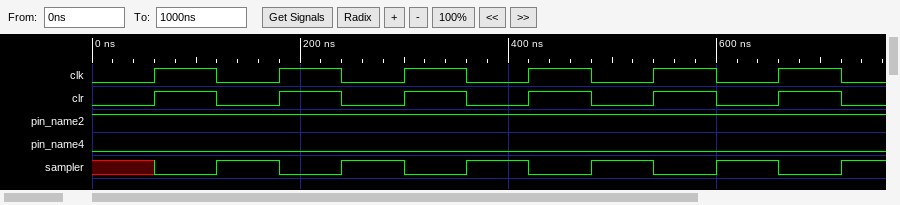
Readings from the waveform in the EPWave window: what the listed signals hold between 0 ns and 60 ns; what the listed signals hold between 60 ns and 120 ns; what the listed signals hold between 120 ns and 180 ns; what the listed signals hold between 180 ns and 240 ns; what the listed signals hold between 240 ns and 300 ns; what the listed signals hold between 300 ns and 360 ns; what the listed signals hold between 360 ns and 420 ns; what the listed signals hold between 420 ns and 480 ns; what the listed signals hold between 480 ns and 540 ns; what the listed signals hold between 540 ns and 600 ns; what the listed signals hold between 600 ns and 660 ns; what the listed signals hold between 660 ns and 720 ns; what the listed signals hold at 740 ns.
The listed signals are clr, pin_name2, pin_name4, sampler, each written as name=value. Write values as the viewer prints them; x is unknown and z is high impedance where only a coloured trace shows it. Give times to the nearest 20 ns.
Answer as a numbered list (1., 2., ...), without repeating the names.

1. clr=0, pin_name2=1, pin_name4=0, sampler=x
2. clr=1, pin_name2=1, pin_name4=0, sampler=0
3. clr=0, pin_name2=1, pin_name4=0, sampler=1
4. clr=1, pin_name2=1, pin_name4=0, sampler=0
5. clr=0, pin_name2=1, pin_name4=0, sampler=1
6. clr=1, pin_name2=1, pin_name4=0, sampler=0
7. clr=0, pin_name2=1, pin_name4=0, sampler=1
8. clr=1, pin_name2=1, pin_name4=0, sampler=0
9. clr=0, pin_name2=1, pin_name4=0, sampler=1
10. clr=1, pin_name2=1, pin_name4=0, sampler=0
11. clr=0, pin_name2=1, pin_name4=0, sampler=1
12. clr=1, pin_name2=1, pin_name4=0, sampler=0
13. clr=0, pin_name2=1, pin_name4=0, sampler=1
